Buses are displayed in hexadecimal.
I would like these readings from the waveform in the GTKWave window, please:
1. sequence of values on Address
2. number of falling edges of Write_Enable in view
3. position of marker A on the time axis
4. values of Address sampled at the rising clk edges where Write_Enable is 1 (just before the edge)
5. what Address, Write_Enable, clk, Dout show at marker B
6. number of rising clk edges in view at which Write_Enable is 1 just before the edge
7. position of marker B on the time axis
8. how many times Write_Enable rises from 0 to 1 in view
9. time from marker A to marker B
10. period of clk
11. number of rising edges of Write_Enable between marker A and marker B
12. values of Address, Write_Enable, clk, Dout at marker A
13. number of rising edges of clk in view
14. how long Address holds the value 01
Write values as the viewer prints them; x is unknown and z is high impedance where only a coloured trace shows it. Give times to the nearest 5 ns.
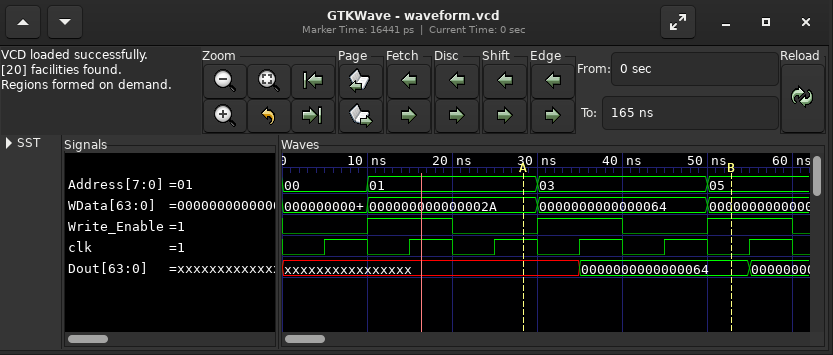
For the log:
00, 01, 03, 05
3
30 ns
01, 03, 05
Address=05, Write_Enable=1, clk=0, Dout=0000000000000064
3
55 ns
3
25 ns
10 ns
2
Address=01, Write_Enable=0, clk=1, Dout=xxxxxxxxxxxxxxxx
6
20 ns
